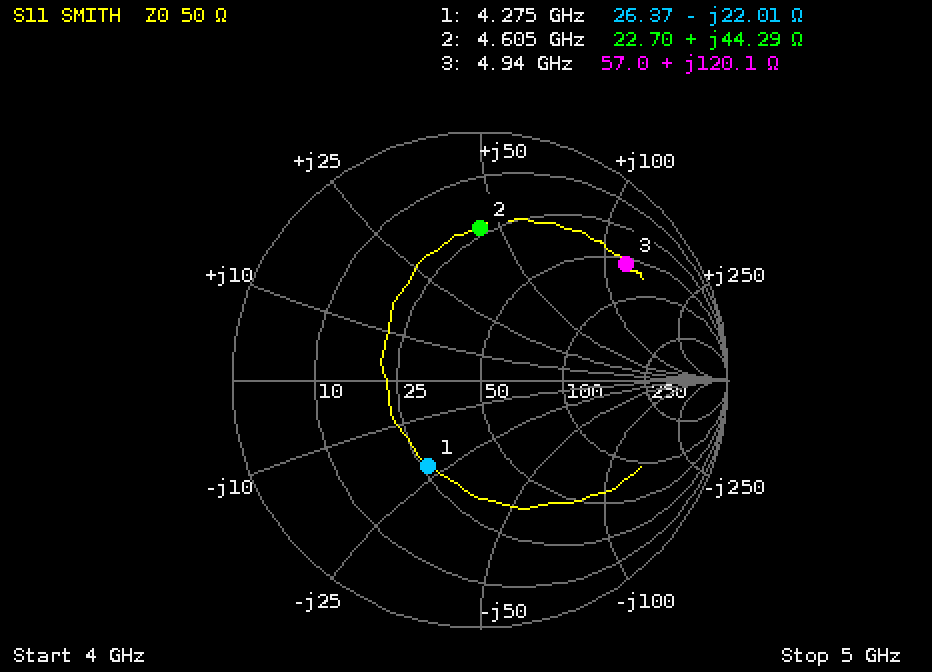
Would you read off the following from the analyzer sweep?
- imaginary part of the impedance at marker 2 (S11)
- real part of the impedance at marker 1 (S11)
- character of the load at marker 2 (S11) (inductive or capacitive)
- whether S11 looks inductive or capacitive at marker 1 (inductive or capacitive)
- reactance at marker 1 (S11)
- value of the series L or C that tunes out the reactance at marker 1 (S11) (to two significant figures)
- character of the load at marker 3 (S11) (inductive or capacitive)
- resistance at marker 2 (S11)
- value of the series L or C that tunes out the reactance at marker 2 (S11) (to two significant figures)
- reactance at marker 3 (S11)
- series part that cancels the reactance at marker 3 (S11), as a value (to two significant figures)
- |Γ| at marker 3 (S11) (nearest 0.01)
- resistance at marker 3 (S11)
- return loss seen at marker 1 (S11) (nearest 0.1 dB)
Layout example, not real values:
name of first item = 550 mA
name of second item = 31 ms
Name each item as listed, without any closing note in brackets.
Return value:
imaginary part of the impedance at marker 2 = +44.29 Ω
real part of the impedance at marker 1 = 26.37 Ω
character of the load at marker 2 (S11) = inductive
whether S11 looks inductive or capacitive at marker 1 = capacitive
reactance at marker 1 = -22.01 Ω
value of the series L or C that tunes out the reactance at marker 1 (S11) = 820 pH
character of the load at marker 3 (S11) = inductive
resistance at marker 2 = 22.70 Ω
value of the series L or C that tunes out the reactance at marker 2 (S11) = 780 fF
reactance at marker 3 = +120.1 Ω
series part that cancels the reactance at marker 3 (S11), as a value = 270 fF
|Γ| at marker 3 (S11) = 0.75
resistance at marker 3 = 57.0 Ω
return loss seen at marker 1 (S11) = 7.8 dB
